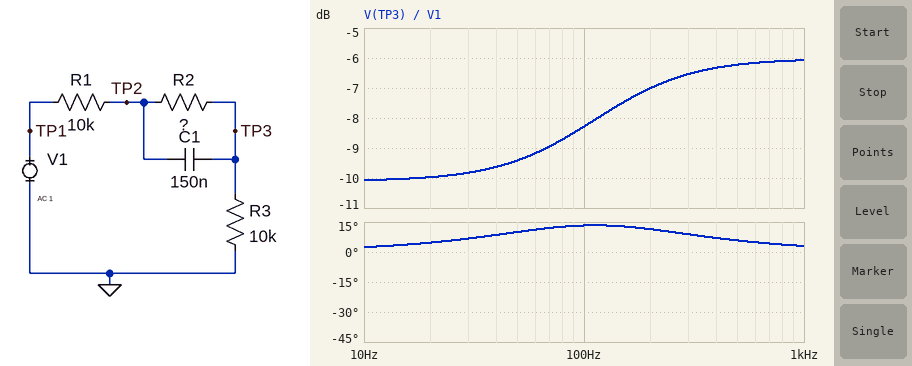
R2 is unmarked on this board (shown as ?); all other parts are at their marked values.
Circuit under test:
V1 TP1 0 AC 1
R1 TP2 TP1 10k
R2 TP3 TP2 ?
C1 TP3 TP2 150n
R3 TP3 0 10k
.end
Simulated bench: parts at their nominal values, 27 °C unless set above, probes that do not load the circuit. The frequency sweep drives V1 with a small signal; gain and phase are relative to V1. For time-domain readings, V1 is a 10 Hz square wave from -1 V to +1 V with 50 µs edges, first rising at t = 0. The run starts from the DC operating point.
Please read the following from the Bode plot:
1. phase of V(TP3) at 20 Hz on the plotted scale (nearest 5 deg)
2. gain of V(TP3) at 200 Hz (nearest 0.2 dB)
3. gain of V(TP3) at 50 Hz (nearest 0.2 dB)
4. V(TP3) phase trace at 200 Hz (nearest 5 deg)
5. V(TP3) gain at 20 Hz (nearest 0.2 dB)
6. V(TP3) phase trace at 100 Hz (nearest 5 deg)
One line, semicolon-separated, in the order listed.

5 deg; -7.0 dB; -9.4 dB; 10 deg; -10.0 dB; 15 deg
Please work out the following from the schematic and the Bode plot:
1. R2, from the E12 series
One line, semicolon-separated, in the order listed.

12 kΩ
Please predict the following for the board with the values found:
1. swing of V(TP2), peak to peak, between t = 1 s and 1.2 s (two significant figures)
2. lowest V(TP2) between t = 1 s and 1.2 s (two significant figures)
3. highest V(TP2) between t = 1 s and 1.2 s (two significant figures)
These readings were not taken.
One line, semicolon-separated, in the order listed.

1.4 V; -690 mV; 690 mV
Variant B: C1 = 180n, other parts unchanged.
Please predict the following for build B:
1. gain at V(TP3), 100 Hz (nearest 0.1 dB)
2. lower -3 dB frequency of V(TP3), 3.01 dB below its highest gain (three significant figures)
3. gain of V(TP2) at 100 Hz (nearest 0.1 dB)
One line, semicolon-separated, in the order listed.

-7.9 dB; 55.1 Hz; -4.2 dB
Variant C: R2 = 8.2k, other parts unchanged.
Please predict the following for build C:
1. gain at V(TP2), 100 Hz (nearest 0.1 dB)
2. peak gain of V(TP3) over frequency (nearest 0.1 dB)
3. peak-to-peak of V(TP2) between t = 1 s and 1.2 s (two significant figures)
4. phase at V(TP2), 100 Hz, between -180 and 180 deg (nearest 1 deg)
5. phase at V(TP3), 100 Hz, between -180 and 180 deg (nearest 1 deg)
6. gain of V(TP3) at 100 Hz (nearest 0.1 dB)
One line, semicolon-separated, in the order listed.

-4.2 dB; -6.0 dB; 1.3 V; -6 deg; 9 deg; -8.1 dB
